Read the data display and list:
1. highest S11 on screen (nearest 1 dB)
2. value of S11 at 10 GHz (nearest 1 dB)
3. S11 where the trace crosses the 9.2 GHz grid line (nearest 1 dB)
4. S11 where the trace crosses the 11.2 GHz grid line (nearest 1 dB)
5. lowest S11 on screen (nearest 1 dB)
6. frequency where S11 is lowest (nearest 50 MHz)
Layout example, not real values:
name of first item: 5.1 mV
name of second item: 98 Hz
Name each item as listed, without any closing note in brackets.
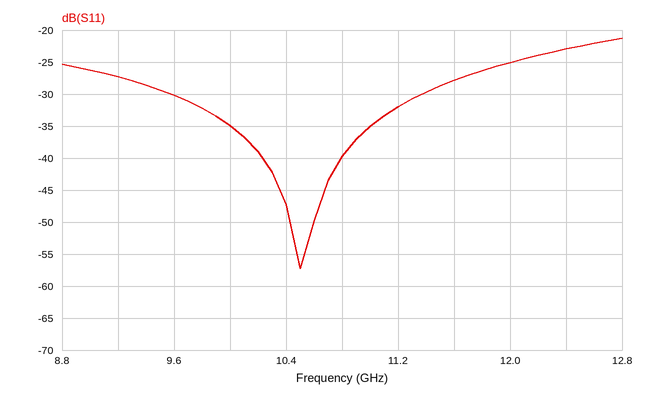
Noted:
highest S11 on screen: -21 dB
value of S11 at 10 GHz: -35 dB
S11 where the trace crosses the 9.2 GHz grid line: -27 dB
S11 where the trace crosses the 11.2 GHz grid line: -32 dB
lowest S11 on screen: -57 dB
frequency where S11 is lowest: 10.50 GHz
